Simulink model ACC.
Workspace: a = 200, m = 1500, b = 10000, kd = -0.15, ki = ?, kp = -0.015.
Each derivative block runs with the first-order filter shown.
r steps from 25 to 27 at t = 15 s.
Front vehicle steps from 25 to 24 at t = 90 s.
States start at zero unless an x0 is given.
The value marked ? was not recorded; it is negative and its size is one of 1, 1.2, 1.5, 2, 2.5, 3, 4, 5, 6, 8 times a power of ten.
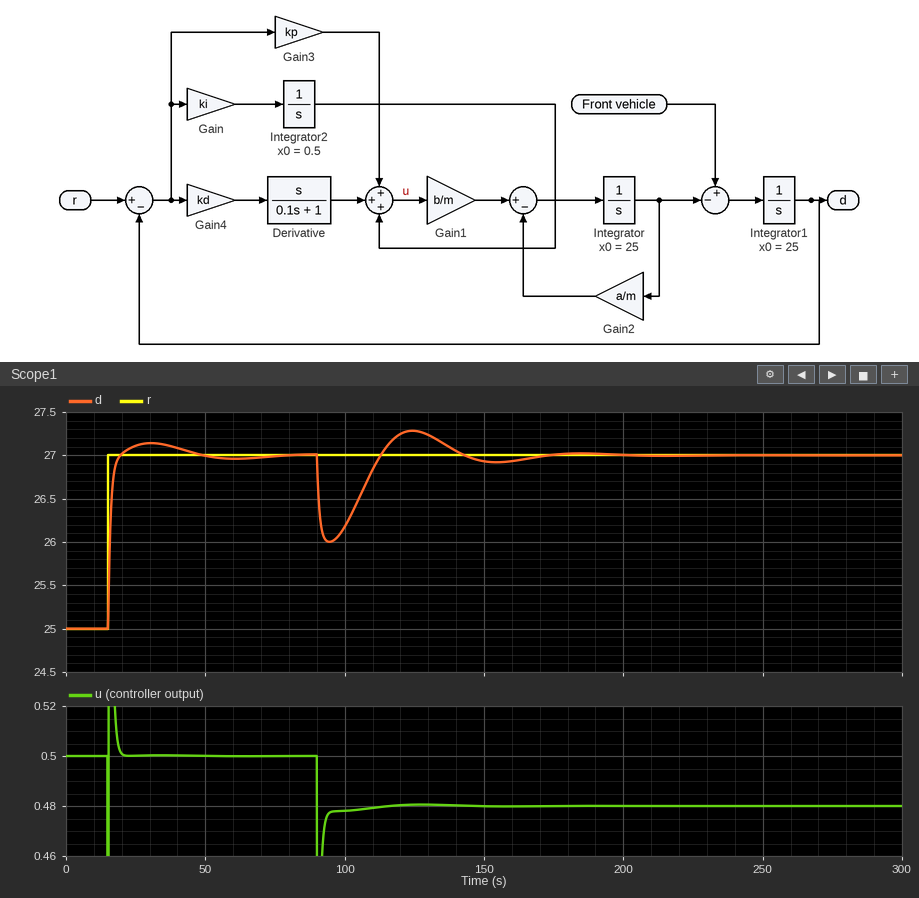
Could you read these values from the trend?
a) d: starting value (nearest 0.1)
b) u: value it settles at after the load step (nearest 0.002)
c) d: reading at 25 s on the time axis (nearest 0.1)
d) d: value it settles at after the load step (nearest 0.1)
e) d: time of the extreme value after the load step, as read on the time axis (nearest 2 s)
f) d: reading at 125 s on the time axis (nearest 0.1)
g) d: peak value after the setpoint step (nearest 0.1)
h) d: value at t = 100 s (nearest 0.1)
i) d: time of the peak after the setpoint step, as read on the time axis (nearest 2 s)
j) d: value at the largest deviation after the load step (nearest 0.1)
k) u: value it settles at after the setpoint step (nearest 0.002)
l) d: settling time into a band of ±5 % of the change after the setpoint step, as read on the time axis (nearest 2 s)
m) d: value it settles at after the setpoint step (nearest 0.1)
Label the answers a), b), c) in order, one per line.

a) 25.0
b) 0.480
c) 27.1
d) 27.0
e) 94 s
f) 27.3
g) 27.1
h) 26.2
i) 30 s
j) 26.0
k) 0.500
l) 38 s
m) 27.0
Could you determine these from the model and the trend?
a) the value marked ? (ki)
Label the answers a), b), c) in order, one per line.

a) -0.002
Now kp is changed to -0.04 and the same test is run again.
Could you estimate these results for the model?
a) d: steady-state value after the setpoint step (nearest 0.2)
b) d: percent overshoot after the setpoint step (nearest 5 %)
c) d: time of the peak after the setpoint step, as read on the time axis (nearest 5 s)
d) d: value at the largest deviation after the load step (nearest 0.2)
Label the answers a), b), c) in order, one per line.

a) 27.0
b) 10 %
c) 20 s
d) 26.2
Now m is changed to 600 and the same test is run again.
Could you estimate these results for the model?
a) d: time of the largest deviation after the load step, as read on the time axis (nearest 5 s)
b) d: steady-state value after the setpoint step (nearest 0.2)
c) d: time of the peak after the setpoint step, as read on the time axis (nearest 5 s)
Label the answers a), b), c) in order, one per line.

a) 100 s
b) 27.0
c) 35 s
